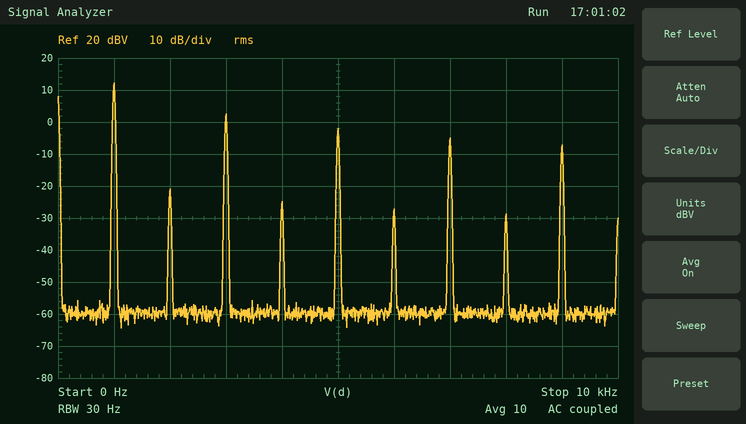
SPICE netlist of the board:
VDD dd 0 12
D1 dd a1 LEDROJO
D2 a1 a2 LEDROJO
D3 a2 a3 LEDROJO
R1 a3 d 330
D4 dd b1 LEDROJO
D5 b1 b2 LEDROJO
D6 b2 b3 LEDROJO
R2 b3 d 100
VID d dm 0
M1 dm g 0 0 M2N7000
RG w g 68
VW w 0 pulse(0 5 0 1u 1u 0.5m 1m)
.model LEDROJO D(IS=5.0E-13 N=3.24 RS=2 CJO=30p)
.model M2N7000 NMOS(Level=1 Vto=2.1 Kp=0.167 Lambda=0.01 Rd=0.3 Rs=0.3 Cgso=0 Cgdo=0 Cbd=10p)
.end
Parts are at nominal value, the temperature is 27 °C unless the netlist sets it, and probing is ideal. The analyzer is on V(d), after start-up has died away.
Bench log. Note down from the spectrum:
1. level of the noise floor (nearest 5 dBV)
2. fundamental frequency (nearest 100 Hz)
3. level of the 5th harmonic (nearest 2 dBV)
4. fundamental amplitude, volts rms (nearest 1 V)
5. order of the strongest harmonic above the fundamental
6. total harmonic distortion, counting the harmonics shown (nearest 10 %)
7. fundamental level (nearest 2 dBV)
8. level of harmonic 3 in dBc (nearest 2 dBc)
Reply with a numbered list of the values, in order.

1. -60 dBV
2. 1.0 kHz
3. -2 dBV
4. 4 V
5. 3
6. 40 %
7. 12 dBV
8. -10 dBc
